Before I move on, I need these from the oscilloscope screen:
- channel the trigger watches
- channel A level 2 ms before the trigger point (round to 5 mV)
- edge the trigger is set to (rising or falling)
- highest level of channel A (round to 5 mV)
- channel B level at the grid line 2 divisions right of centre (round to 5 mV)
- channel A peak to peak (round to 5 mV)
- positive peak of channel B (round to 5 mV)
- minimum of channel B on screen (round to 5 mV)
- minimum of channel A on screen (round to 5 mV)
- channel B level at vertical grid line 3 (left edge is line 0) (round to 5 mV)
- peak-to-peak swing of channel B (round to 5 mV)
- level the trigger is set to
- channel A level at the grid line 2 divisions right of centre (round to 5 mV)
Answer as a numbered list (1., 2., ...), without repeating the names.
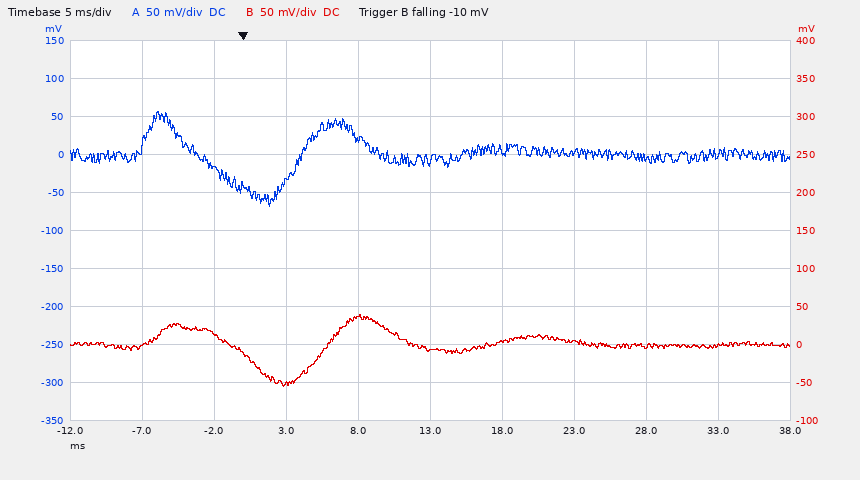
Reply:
1. channel B
2. -15 mV
3. falling
4. 55 mV
5. 5 mV
6. 125 mV
7. 40 mV
8. -55 mV
9. -70 mV
10. -50 mV
11. 95 mV
12. -10 mV
13. 5 mV
